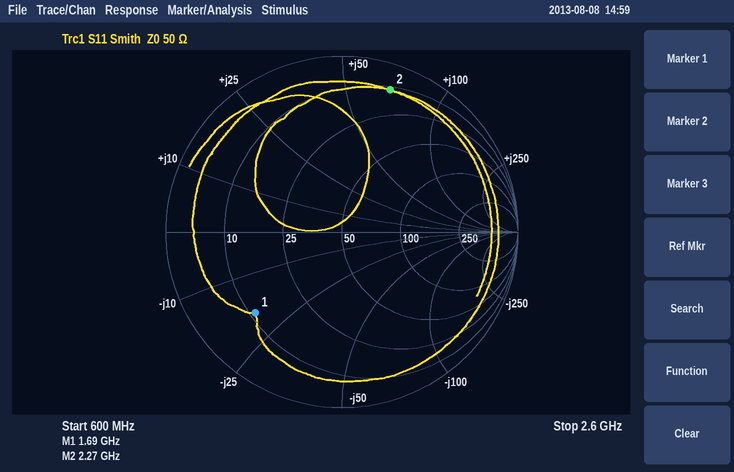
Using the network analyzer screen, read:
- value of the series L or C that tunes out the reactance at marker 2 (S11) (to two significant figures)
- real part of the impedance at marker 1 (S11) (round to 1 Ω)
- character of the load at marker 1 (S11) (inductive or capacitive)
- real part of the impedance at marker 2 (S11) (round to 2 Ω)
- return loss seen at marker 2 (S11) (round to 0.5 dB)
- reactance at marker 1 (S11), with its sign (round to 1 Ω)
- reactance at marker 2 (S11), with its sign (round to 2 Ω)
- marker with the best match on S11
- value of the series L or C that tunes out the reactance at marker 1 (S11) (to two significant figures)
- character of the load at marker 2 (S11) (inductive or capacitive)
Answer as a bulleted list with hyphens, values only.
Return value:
- 1.0 pF
- 11 Ω
- capacitive
- 12 Ω
- 1.5 dB
- -19 Ω
- +68 Ω
- marker 1
- 1.8 nH
- inductive
